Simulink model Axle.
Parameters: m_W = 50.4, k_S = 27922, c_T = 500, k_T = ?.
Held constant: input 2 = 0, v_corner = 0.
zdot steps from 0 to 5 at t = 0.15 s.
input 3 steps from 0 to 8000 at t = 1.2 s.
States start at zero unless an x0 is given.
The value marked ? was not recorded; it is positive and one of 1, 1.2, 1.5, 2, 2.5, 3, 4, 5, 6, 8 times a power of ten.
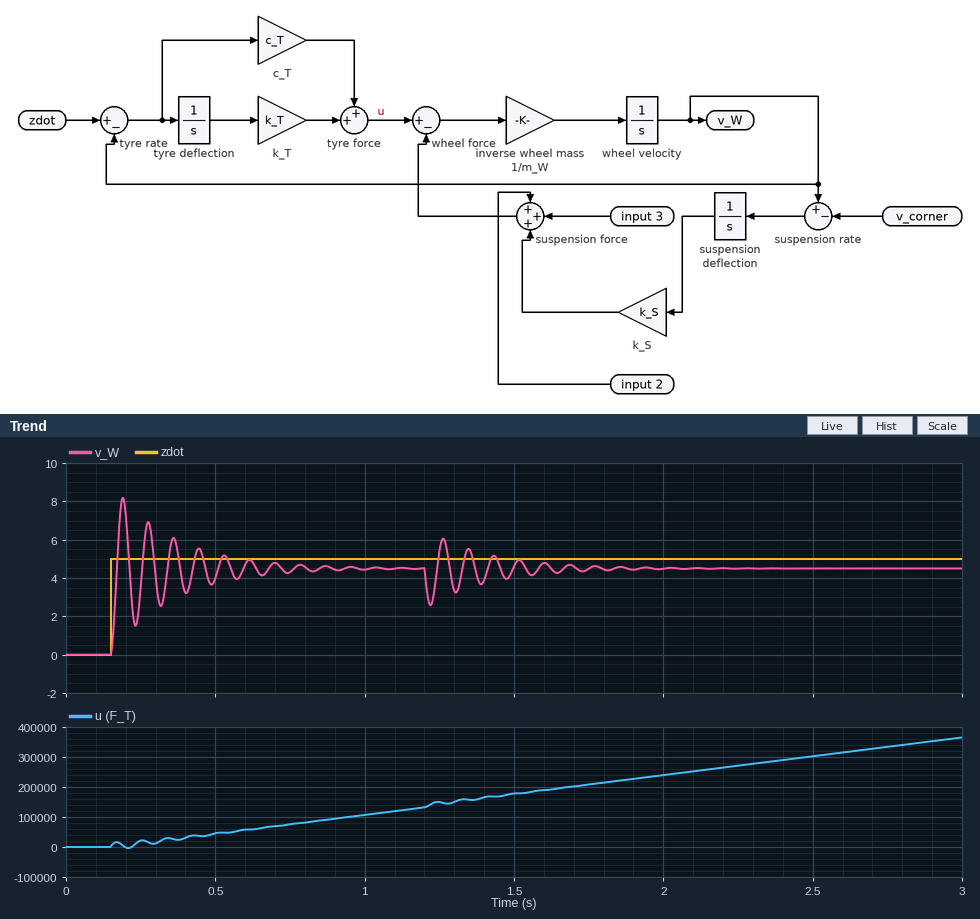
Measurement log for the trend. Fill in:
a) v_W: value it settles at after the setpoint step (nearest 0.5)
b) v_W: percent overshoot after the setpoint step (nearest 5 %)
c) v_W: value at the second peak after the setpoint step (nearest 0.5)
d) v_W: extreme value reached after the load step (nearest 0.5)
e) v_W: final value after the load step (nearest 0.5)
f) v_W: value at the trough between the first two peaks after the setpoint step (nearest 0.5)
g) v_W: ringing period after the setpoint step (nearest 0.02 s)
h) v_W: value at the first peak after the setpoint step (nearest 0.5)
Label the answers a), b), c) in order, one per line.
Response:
a) 4.5
b) 80 %
c) 7.0
d) 2.5
e) 4.5
f) 1.5
g) 0.08 s
h) 8.0
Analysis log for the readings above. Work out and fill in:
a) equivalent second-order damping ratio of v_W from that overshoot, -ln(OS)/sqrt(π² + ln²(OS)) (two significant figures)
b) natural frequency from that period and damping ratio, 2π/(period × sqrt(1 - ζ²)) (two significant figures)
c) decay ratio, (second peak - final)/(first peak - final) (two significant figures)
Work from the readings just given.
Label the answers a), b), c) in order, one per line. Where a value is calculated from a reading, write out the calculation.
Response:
a) ln(0.8) = -0.223; 0.223 / sqrt(9.870 + 0.050) = 0.071
b) 2π / (0.08 × sqrt(1 - 0.071²)) = 79 rad/s
c) (7 - 4.5) / (8 - 4.5) = 0.71
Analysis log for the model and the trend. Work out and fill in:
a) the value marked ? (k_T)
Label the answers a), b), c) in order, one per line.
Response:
a) 250000
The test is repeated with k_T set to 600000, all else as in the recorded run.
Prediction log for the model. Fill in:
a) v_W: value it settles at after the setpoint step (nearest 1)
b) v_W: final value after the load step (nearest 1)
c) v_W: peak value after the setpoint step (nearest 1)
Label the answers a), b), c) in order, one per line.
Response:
a) 5
b) 5
c) 9
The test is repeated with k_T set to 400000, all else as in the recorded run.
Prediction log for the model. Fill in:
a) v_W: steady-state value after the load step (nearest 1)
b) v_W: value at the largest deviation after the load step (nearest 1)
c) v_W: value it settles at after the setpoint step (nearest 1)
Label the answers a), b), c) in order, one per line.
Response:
a) 5
b) 3
c) 5
